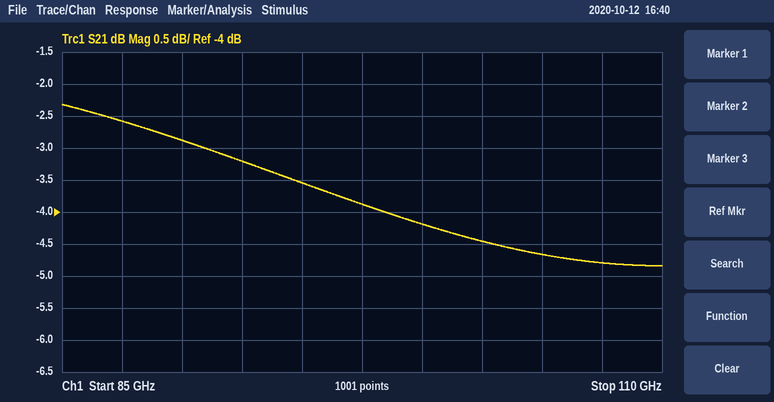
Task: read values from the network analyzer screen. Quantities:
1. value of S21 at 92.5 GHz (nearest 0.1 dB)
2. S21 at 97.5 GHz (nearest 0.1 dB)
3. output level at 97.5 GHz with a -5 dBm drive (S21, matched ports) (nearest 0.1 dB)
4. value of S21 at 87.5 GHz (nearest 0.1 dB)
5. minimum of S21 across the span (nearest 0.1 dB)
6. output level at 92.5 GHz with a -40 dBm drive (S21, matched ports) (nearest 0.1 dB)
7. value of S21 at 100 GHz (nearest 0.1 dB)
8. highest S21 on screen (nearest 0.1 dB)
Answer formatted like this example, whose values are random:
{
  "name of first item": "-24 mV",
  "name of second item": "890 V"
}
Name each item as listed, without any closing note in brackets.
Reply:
{
  "value of S21 at 92.5 GHz": "-3.2 dB",
  "S21 at 97.5 GHz": "-3.9 dB",
  "output level at 97.5 GHz with a -5 dBm drive (S21, matched ports)": "-8.9 dBm",
  "value of S21 at 87.5 GHz": "-2.6 dB",
  "minimum of S21 across the span": "-4.8 dB",
  "output level at 92.5 GHz with a -40 dBm drive (S21, matched ports)": "-43.2 dBm",
  "value of S21 at 100 GHz": "-4.2 dB",
  "highest S21 on screen": "-2.3 dB"
}
